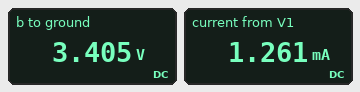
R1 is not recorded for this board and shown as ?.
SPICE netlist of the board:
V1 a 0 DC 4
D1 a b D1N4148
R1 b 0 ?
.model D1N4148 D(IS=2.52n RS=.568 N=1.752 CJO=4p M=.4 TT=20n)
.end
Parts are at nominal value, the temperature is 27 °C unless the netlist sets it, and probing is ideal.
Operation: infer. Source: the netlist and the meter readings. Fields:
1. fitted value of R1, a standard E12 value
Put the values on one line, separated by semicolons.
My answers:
2.7 kΩ
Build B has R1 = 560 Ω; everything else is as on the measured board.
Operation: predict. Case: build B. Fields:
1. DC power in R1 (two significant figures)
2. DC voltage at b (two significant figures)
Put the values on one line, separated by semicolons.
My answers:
20 mW; 3.3 V
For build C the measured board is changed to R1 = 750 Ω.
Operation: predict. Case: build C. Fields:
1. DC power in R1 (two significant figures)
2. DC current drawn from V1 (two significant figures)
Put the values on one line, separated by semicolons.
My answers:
15 mW; 4.5 mA
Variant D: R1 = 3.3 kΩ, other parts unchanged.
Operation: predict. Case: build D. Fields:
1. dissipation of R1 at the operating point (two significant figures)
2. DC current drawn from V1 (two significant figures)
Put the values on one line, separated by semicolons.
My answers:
3.5 mW; 1.0 mA
